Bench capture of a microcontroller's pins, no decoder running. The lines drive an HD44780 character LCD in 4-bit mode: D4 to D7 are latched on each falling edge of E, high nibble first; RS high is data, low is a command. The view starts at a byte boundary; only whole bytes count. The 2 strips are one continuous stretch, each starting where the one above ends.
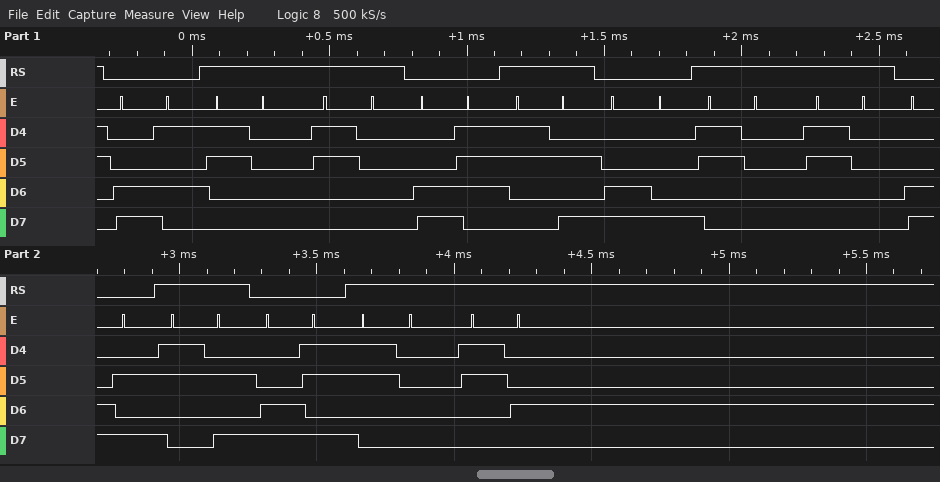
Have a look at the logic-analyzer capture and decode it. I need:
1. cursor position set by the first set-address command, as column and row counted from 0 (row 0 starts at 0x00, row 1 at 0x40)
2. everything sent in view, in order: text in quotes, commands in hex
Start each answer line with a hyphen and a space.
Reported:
- column 5, row 1
- 0xC5 "00" 0xC7 ":" 0xC8 "00" 0xCA ":" 0xCB "04"
